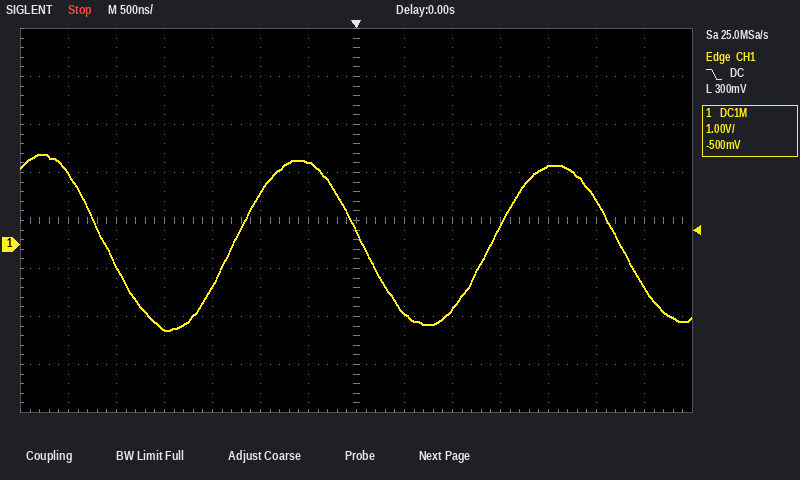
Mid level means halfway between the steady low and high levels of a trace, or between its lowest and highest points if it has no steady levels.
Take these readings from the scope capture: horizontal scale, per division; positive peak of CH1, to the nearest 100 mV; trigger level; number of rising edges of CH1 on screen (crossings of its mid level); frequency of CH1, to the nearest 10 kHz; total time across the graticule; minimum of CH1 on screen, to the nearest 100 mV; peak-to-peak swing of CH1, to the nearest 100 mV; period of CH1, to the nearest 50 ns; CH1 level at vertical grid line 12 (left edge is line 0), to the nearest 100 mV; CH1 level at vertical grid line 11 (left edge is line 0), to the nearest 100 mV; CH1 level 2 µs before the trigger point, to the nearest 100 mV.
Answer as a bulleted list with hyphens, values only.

- 500 ns
- 1.9 V
- 300 mV
- 2
- 370 kHz
- 7 µs
- -1.8 V
- 3.7 V
- 2.70 µs
- 900 mV
- 1.6 V
- -1.8 V
